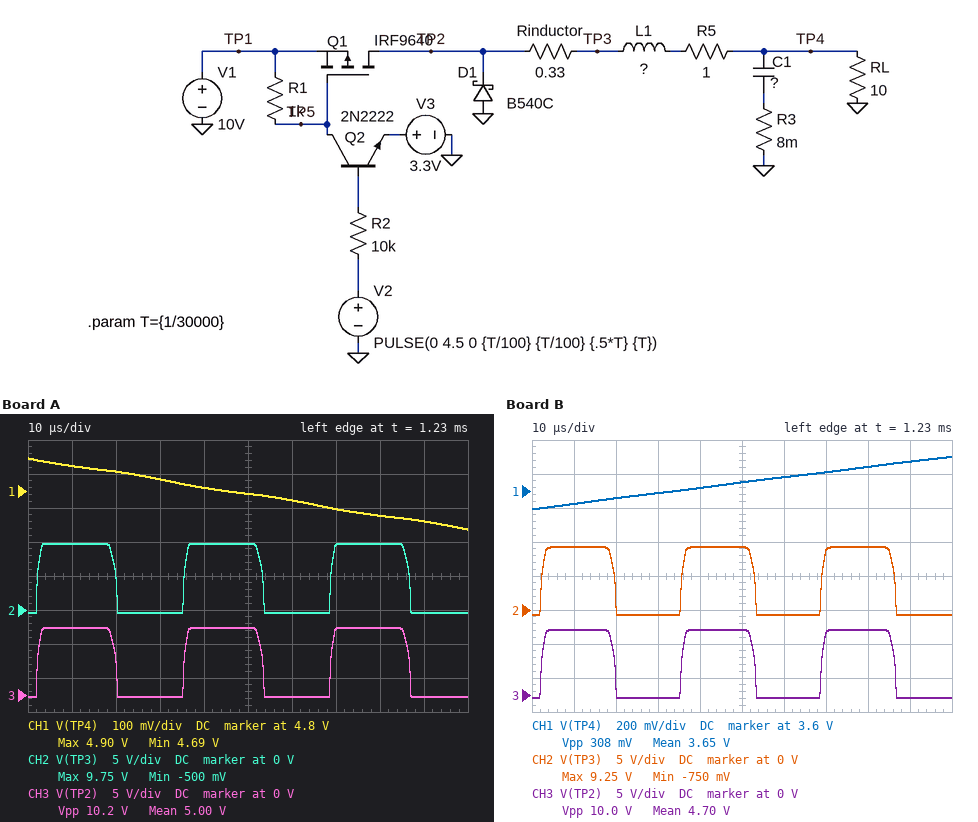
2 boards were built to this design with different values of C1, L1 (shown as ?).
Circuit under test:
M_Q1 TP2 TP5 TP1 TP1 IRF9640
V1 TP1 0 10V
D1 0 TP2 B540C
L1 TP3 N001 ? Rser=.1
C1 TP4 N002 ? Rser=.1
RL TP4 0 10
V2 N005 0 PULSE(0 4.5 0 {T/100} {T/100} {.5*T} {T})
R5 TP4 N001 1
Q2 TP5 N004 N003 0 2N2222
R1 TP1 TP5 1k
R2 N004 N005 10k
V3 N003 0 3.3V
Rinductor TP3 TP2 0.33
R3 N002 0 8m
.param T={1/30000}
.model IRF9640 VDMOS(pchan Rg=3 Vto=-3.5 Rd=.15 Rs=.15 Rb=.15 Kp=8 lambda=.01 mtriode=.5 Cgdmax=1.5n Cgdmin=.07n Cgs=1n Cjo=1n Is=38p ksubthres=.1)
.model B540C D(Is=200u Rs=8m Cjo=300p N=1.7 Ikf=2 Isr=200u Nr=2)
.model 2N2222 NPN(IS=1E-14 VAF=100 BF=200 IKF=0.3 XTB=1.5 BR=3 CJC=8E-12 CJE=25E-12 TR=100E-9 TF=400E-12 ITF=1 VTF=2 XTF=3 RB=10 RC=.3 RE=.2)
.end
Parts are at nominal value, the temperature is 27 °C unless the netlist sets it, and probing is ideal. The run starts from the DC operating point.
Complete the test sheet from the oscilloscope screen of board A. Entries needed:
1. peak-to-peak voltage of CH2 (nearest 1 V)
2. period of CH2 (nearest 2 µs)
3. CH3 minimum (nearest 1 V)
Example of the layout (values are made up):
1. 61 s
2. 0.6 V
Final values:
1. 10 V
2. 34 µs
3. 0 V
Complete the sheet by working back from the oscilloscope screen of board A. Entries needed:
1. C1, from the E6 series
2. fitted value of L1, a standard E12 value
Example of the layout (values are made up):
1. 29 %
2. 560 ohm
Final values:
1. 47 µF
2. 1.8 mH
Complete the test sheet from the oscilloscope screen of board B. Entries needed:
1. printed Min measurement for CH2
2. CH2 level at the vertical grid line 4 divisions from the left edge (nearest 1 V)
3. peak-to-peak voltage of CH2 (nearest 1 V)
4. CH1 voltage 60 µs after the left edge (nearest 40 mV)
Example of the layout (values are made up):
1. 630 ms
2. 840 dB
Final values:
1. -750 mV
2. 9 V
3. 10 V
4. 3.68 V
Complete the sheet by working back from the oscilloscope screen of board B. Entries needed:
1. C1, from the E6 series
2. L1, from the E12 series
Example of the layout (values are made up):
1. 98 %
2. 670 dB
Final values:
1. 220 µF
2. 2.7 mH
